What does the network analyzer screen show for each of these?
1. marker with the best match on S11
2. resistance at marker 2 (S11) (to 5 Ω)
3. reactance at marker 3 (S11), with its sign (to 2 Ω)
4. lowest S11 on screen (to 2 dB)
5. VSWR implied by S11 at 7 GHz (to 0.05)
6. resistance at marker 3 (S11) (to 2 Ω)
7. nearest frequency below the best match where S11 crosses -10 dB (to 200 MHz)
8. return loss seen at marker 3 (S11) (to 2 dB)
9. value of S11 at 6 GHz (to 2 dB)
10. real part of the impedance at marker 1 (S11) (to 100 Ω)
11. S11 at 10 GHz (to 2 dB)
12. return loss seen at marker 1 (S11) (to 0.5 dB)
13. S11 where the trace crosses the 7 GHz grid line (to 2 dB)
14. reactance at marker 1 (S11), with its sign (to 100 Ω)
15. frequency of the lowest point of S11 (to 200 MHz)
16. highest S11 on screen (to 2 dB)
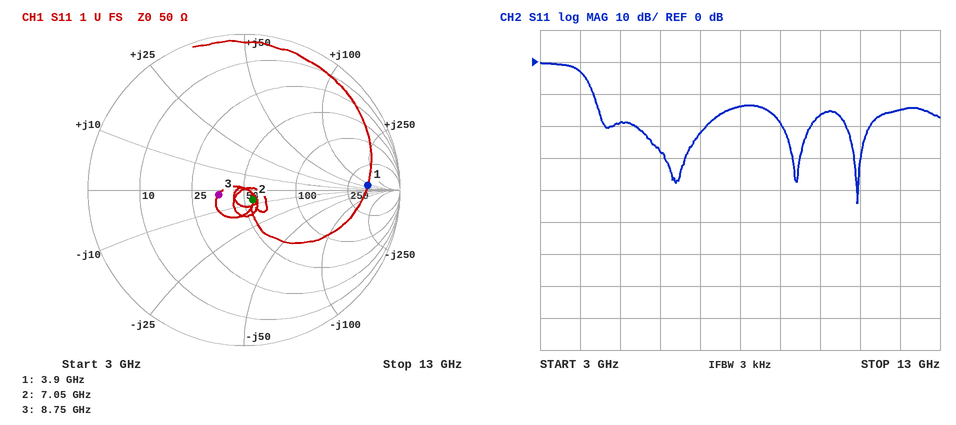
marker 2
55 Ω
-2 Ω
-44 dB
1.15
36 Ω
4.4 GHz
16 dB
-28 dB
400 Ω
-16 dB
2.0 dB
-22 dB
+100 Ω
11.0 GHz
0 dB
